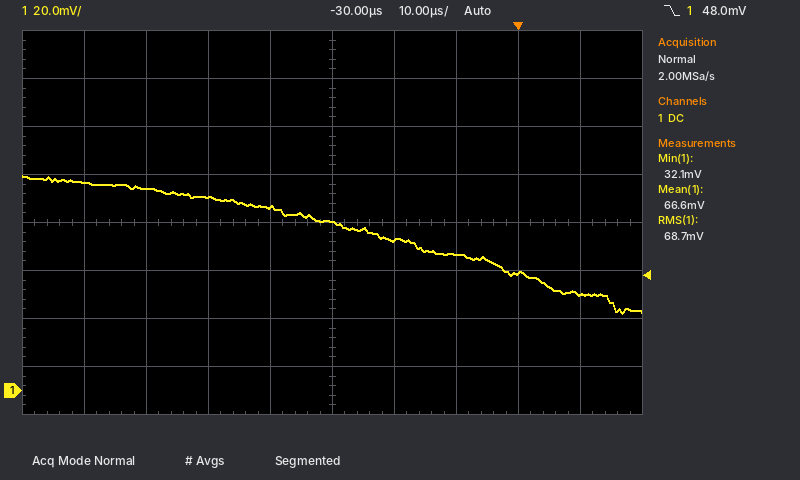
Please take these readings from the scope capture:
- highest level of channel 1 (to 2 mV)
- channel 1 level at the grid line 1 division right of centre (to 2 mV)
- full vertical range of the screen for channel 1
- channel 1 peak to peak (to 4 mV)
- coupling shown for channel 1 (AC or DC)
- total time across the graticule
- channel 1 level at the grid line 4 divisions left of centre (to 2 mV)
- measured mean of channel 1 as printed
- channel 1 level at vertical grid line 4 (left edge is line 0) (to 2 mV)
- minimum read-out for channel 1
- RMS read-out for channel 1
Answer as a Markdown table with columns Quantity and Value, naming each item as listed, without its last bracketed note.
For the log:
| Quantity | Value |
|---|---|
| highest level of channel 1 | 90 mV |
| channel 1 level at the grid line 1 division right of centre | 62 mV |
| full vertical range of the screen for channel 1 | 160 mV |
| channel 1 peak to peak | 56 mV |
| coupling shown for channel 1 | DC |
| total time across the graticule | 100 µs |
| channel 1 level at the grid line 4 divisions left of centre | 86 mV |
| measured mean of channel 1 as printed | 66.6 mV |
| channel 1 level at vertical grid line 4 (left edge is line 0) | 76 mV |
| minimum read-out for channel 1 | 32.1 mV |
| RMS read-out for channel 1 | 68.7 mV |
